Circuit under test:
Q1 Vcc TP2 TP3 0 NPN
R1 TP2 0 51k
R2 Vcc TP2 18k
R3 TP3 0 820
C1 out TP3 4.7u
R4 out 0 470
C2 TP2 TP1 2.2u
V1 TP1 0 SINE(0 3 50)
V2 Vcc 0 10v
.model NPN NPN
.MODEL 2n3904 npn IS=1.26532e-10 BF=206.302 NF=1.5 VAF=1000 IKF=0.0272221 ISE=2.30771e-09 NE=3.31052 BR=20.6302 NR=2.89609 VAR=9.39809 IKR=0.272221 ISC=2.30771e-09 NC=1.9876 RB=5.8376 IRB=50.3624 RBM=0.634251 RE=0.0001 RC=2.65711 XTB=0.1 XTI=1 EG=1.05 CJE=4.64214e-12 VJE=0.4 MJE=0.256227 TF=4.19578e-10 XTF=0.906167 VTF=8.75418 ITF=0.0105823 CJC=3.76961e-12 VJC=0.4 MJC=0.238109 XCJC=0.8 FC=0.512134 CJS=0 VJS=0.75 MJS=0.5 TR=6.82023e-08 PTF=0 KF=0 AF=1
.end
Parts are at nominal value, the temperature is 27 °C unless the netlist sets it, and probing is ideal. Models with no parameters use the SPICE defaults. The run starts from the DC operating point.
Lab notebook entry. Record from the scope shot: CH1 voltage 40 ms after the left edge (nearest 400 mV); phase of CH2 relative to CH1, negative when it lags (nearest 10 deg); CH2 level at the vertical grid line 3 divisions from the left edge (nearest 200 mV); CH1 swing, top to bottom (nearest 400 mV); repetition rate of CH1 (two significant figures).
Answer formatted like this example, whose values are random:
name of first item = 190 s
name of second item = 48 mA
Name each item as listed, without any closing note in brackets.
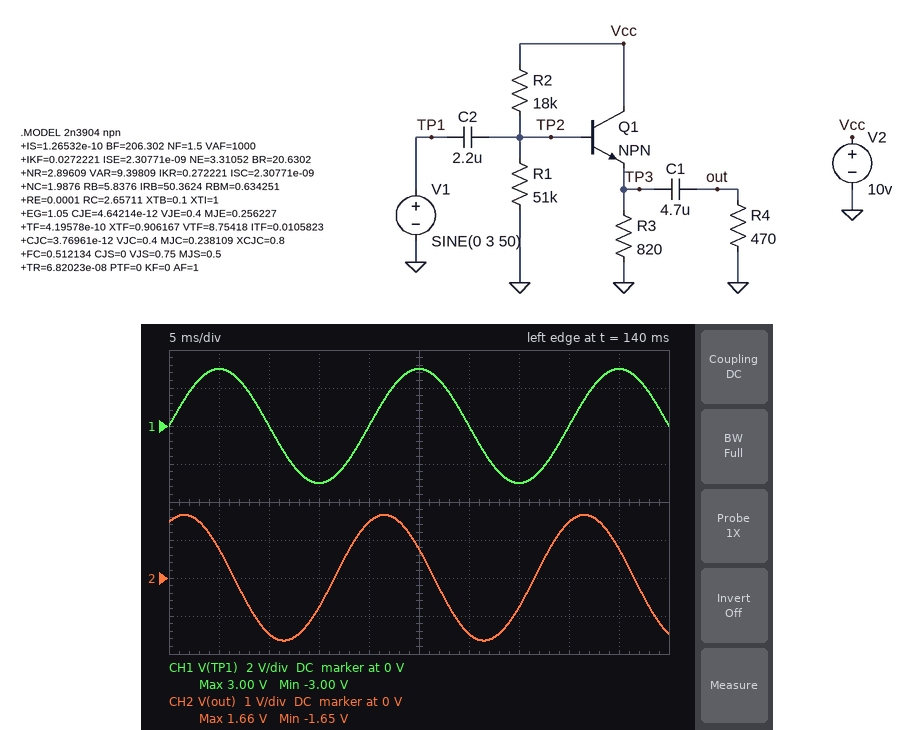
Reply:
CH1 voltage 40 ms after the left edge = 0 V
phase of CH2 relative to CH1, negative when it lags = 60 deg
CH2 level at the vertical grid line 3 divisions from the left edge = -800 mV
CH1 swing, top to bottom = 6.0 V
repetition rate of CH1 = 50 Hz
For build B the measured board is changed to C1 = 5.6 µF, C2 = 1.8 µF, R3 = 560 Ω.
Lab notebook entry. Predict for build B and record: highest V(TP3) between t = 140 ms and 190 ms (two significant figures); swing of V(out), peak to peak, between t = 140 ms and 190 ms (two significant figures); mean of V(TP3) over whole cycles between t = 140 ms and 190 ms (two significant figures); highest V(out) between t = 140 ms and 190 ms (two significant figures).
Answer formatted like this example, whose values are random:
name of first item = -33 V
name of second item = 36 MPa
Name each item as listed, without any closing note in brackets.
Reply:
highest V(TP3) between t = 140 ms and 190 ms = 8.2 V
swing of V(out), peak to peak, between t = 140 ms and 190 ms = 3.7 V
mean of V(TP3) over whole cycles between t = 140 ms and 190 ms = 5.3 V
highest V(out) between t = 140 ms and 190 ms = 1.8 V
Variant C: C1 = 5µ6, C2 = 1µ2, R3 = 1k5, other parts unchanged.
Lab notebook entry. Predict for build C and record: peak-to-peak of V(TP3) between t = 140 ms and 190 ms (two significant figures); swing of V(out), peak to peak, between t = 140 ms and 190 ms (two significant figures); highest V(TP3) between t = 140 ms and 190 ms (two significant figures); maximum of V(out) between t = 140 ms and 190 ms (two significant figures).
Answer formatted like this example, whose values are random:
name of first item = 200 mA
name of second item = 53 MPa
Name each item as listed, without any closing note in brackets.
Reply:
peak-to-peak of V(TP3) between t = 140 ms and 190 ms = 5.5 V
swing of V(out), peak to peak, between t = 140 ms and 190 ms = 3.4 V
highest V(TP3) between t = 140 ms and 190 ms = 8.9 V
maximum of V(out) between t = 140 ms and 190 ms = 1.8 V
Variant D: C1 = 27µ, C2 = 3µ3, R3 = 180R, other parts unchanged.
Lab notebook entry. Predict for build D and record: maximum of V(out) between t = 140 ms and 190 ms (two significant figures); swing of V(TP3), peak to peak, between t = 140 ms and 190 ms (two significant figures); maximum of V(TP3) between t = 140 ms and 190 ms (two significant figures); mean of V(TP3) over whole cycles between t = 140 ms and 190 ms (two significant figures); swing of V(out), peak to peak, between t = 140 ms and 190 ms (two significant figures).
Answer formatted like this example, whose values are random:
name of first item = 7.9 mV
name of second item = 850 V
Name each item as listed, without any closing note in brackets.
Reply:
maximum of V(out) between t = 140 ms and 190 ms = 2.8 V
swing of V(TP3), peak to peak, between t = 140 ms and 190 ms = 5.7 V
maximum of V(TP3) between t = 140 ms and 190 ms = 6.7 V
mean of V(TP3) over whole cycles between t = 140 ms and 190 ms = 3.8 V
swing of V(out), peak to peak, between t = 140 ms and 190 ms = 5.6 V
